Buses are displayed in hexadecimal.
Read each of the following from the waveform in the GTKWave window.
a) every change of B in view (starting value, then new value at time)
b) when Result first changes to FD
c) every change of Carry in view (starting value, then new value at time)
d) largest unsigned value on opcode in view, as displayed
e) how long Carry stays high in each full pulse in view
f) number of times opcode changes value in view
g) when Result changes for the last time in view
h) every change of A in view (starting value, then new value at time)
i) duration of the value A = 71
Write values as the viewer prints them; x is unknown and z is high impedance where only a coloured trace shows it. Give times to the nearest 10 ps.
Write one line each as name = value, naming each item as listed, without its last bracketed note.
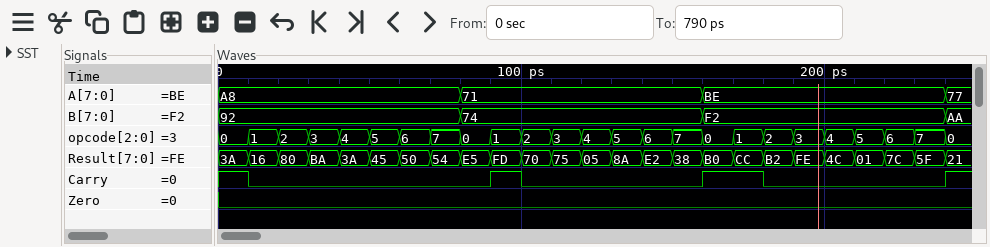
every change of B in view = 92, 74 at 80 ps, F2 at 160 ps, AA at 240 ps
when Result first changes to FD = 90 ps
every change of Carry in view = 1, 0 at 10 ps, 1 at 90 ps, 0 at 100 ps, 1 at 160 ps, 0 at 180 ps, 1 at 240 ps
largest unsigned value on opcode in view, as displayed = 7
how long Carry stays high in each full pulse in view = 10 ps, 20 ps
number of times opcode changes value in view = 24
when Result changes for the last time in view = 240 ps
every change of A in view = A8, 71 at 80 ps, BE at 160 ps, 77 at 240 ps
duration of the value A = 71 = 80 ps
